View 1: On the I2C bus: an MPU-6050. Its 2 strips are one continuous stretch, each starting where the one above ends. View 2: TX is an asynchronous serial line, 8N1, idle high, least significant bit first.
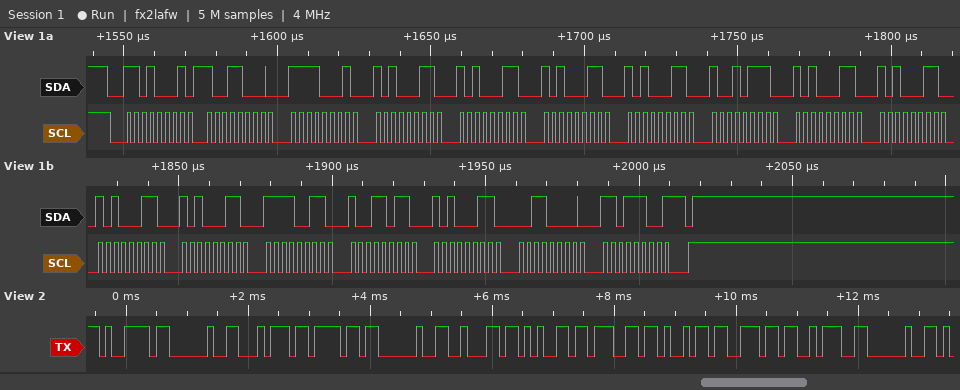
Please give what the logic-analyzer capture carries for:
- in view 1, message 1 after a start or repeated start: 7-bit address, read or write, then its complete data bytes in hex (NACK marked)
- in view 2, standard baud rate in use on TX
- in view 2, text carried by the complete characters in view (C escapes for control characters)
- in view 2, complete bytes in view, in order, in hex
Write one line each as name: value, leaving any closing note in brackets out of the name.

in view 1, message 1 after a start or repeated start: 7-bit address, read or write, then its complete data bytes in hex: 0x68 read: 98 F1 A3 A3 A3 A3 97 A3 A3 A3 A3 F3 9B A3 30 DC NACK
in view 2, standard baud rate in use on TX: 9600 baud
in view 2, text carried by the complete characters in view: "y to begin: "
in view 2, complete bytes in view, in order, in hex: 79 20 74 6F 20 62 65 67 69 6E 3A 20
